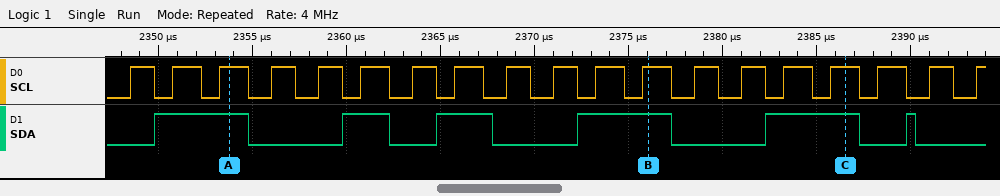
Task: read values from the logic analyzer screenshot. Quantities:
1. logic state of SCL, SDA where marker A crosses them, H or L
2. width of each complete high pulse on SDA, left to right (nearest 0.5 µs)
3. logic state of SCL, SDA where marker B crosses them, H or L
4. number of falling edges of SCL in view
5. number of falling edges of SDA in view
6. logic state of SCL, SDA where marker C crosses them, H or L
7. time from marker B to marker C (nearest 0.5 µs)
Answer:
SCL=H, SDA=H
5 µs, 2.5 µs, 3 µs, 5 µs, 5 µs, 0.5 µs
SCL=H, SDA=H
18
6
SCL=H, SDA=H
10.5 µs
